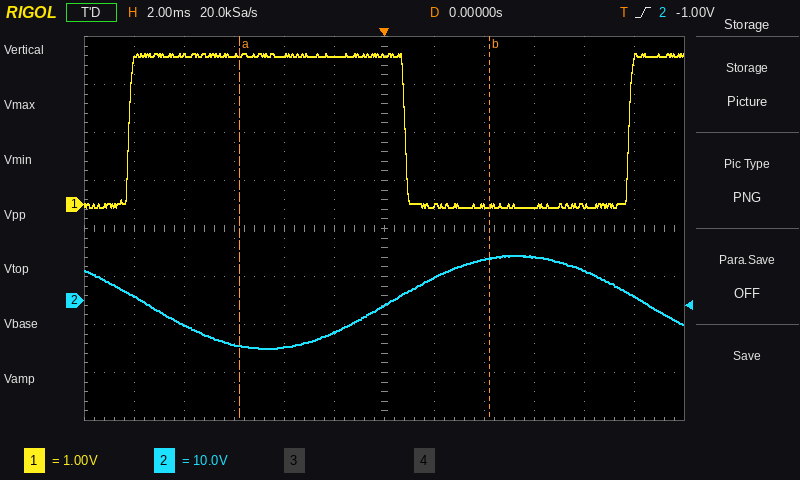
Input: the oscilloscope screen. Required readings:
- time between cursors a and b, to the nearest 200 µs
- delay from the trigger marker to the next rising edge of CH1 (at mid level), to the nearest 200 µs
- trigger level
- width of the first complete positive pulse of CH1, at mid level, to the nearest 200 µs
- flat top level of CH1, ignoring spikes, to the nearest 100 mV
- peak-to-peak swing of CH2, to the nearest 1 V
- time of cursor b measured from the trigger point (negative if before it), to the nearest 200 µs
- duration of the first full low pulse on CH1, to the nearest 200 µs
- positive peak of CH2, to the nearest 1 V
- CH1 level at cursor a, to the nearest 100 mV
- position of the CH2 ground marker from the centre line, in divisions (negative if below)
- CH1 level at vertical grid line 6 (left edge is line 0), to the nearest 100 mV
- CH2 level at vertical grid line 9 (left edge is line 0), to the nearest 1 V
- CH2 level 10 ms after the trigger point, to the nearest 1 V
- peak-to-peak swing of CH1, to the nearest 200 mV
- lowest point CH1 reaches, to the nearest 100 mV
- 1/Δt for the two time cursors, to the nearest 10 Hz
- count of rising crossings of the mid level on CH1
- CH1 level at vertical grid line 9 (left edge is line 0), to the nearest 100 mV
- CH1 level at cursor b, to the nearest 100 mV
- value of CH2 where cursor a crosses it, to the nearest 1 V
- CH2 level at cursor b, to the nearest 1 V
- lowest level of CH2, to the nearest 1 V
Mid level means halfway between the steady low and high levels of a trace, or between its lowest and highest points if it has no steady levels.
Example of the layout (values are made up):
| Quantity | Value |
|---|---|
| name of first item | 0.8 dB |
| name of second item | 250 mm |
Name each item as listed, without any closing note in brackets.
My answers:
| Quantity | Value |
|---|---|
| time between cursors a and b, to the nearest 200 µs | 10.0 ms |
| delay from the trigger marker to the next rising edge of CH1 (at mid level), to the nearest 200 µs | 9.8 ms |
| trigger level | -1.00 V |
| width of the first complete positive pulse of CH1, at mid level, to the nearest 200 µs | 11.0 ms |
| flat top level of CH1, ignoring spikes, to the nearest 100 mV | 3.1 V |
| peak-to-peak swing of CH2, to the nearest 1 V | 19 V |
| time of cursor b measured from the trigger point (negative if before it), to the nearest 200 µs | +4.2 ms |
| duration of the first full low pulse on CH1, to the nearest 200 µs | 9.0 ms |
| positive peak of CH2, to the nearest 1 V | 9 V |
| CH1 level at cursor a, to the nearest 100 mV | 3.1 V |
| position of the CH2 ground marker from the centre line, in divisions | -1.5 div |
| CH1 level at vertical grid line 6 (left edge is line 0), to the nearest 100 mV | 3.1 V |
| CH2 level at vertical grid line 9 (left edge is line 0), to the nearest 1 V | 9 V |
| CH2 level 10 ms after the trigger point, to the nearest 1 V | 1 V |
| peak-to-peak swing of CH1, to the nearest 200 mV | 3.2 V |
| lowest point CH1 reaches, to the nearest 100 mV | -100 mV |
| 1/Δt for the two time cursors, to the nearest 10 Hz | 100 Hz |
| count of rising crossings of the mid level on CH1 | 2 |
| CH1 level at vertical grid line 9 (left edge is line 0), to the nearest 100 mV | -100 mV |
| CH1 level at cursor b, to the nearest 100 mV | 0.0 V |
| value of CH2 where cursor a crosses it, to the nearest 1 V | -9 V |
| CH2 level at cursor b, to the nearest 1 V | 9 V |
| lowest level of CH2, to the nearest 1 V | -10 V |
